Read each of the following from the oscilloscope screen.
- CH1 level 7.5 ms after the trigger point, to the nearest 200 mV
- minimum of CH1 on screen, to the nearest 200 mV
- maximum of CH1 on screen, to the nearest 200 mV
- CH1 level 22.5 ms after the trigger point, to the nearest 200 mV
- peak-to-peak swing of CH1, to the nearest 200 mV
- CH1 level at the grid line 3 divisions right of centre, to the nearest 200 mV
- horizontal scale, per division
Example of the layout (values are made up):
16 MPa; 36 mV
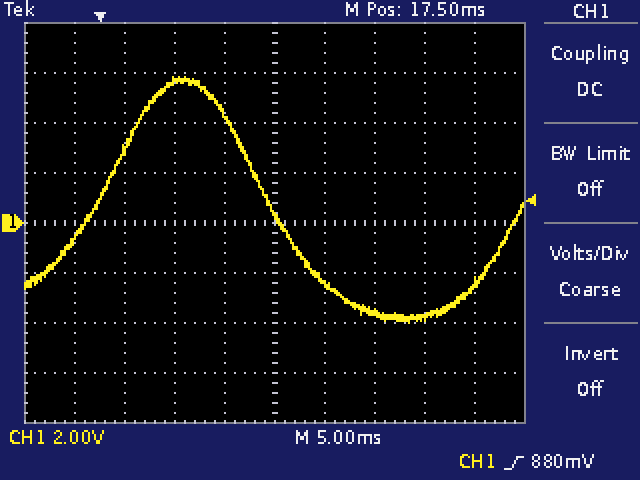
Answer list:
5.6 V; -4.0 V; 5.8 V; -2.4 V; 9.8 V; -3.8 V; 5 ms
